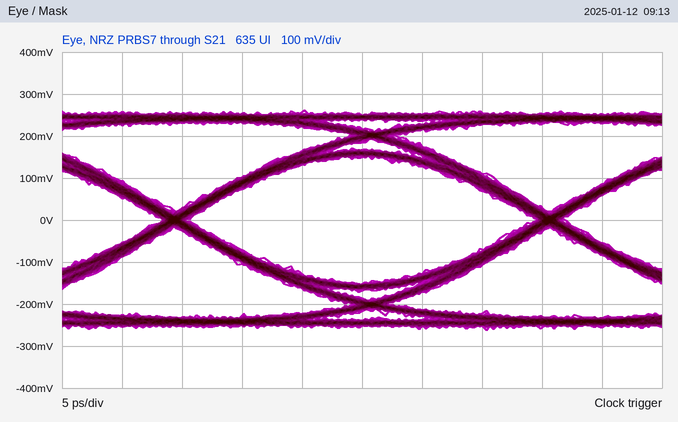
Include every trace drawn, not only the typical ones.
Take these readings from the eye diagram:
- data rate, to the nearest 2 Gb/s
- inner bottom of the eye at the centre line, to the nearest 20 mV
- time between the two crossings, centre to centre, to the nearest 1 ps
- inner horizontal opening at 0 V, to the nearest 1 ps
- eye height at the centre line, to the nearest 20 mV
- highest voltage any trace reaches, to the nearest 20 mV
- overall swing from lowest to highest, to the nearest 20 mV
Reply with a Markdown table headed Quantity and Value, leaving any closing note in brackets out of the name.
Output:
| Quantity | Value |
|---|---|
| data rate, to the nearest 2 Gb/s | 32 Gb/s |
| inner bottom of the eye at the centre line, to the nearest 20 mV | -160 mV |
| time between the two crossings, centre to centre, to the nearest 1 ps | 31 ps |
| inner horizontal opening at 0 V, to the nearest 1 ps | 29 ps |
| eye height at the centre line, to the nearest 20 mV | 300 mV |
| highest voltage any trace reaches, to the nearest 20 mV | 260 mV |
| overall swing from lowest to highest, to the nearest 20 mV | 520 mV |
